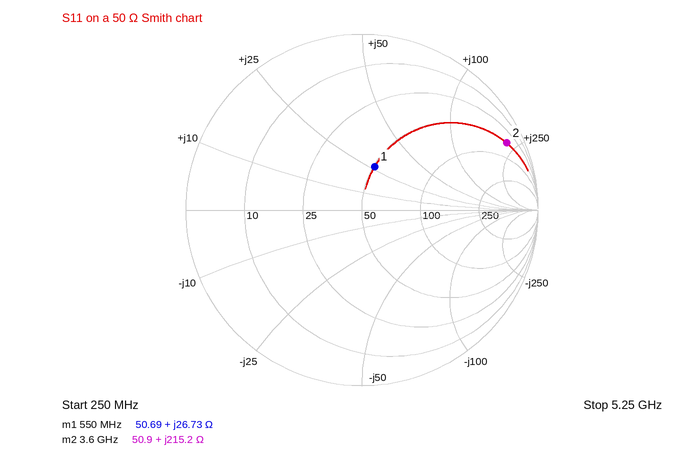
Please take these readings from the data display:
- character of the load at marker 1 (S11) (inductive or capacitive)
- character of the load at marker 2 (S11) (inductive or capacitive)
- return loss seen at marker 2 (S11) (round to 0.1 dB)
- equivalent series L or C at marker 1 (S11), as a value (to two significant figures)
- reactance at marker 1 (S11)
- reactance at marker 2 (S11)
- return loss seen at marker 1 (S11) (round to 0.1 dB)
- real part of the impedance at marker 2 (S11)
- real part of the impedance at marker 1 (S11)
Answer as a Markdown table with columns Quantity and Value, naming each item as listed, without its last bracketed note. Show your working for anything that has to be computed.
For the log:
| Quantity | Value |
|---|---|
| character of the load at marker 1 (S11) | inductive |
| character of the load at marker 2 (S11) | inductive |
| return loss seen at marker 2 (S11) | 0.9 dB |
| equivalent series L or C at marker 1 (S11), as a value | L = 26.73 Ω/(2π × 550 MHz) ≈ 7.7 nH |
| reactance at marker 1 | +26.73 Ω |
| reactance at marker 2 | +215.2 Ω |
| return loss seen at marker 1 (S11) | 11.8 dB |
| real part of the impedance at marker 2 | 50.9 Ω |
| real part of the impedance at marker 1 | 50.69 Ω |
